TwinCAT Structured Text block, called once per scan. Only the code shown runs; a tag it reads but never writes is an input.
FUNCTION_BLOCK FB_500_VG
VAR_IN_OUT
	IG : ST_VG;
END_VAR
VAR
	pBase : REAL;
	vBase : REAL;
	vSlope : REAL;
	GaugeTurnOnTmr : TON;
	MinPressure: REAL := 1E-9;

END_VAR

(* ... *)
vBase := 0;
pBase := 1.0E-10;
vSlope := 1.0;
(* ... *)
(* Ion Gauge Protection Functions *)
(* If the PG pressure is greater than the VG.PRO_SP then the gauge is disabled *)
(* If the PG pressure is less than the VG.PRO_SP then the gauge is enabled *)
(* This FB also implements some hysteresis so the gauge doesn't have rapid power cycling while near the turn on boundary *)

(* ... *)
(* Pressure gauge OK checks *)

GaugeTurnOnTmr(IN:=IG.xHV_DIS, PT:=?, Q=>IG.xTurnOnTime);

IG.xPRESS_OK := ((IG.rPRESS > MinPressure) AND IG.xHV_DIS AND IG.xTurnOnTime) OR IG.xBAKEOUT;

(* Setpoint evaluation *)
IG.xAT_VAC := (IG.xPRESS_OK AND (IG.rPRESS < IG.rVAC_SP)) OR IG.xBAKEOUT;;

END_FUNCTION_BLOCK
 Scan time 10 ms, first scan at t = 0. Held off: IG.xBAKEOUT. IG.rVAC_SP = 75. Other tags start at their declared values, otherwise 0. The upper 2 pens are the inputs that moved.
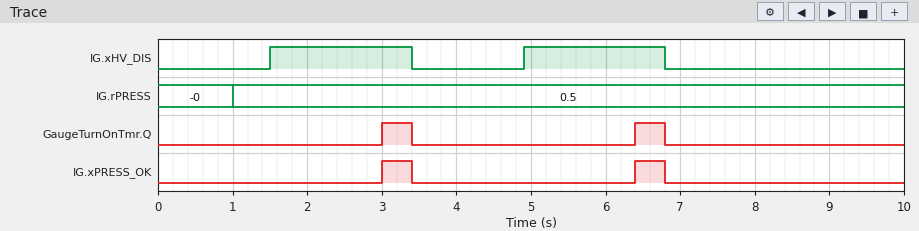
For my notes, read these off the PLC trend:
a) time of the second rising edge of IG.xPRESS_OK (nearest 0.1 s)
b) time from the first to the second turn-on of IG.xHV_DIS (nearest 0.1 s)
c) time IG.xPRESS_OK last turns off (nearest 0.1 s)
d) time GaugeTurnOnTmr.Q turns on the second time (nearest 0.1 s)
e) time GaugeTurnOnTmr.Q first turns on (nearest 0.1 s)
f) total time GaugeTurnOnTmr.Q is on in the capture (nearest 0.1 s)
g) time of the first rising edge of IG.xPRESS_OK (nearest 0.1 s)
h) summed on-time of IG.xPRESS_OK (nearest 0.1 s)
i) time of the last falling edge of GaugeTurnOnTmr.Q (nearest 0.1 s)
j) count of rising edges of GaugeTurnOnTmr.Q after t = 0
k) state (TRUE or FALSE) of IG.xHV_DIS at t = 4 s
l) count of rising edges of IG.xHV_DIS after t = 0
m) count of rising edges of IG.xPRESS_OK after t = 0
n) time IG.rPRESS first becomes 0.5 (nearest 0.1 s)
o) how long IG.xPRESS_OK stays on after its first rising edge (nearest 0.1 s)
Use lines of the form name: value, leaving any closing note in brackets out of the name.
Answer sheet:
time of the second rising edge of IG.xPRESS_OK: 6.4 s
time from the first to the second turn-on of IG.xHV_DIS: 3.4 s
time IG.xPRESS_OK last turns off: 6.8 s
time GaugeTurnOnTmr.Q turns on the second time: 6.4 s
time GaugeTurnOnTmr.Q first turns on: 3.0 s
total time GaugeTurnOnTmr.Q is on in the capture: 0.8 s
time of the first rising edge of IG.xPRESS_OK: 3.0 s
summed on-time of IG.xPRESS_OK: 0.8 s
time of the last falling edge of GaugeTurnOnTmr.Q: 6.8 s
count of rising edges of GaugeTurnOnTmr.Q after t = 0: 2
state (TRUE or FALSE) of IG.xHV_DIS at t = 4 s: FALSE
count of rising edges of IG.xHV_DIS after t = 0: 2
count of rising edges of IG.xPRESS_OK after t = 0: 2
time IG.rPRESS first becomes 0.5: 1.0 s
how long IG.xPRESS_OK stays on after its first rising edge: 0.4 s
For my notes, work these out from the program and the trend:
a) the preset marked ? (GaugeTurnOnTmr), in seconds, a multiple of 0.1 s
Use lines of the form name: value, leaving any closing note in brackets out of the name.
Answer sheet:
the preset marked ? (GaugeTurnOnTmr), in seconds, a multiple of 0.1 s: 1.5 s
